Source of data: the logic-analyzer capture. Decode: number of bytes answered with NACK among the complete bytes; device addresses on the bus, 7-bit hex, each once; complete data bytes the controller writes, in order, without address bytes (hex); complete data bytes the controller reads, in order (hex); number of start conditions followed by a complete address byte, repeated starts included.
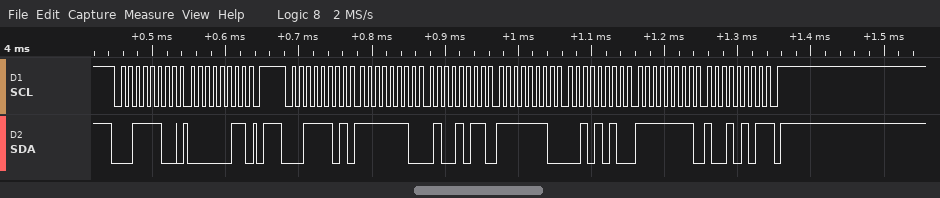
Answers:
1
0x1E
03
FE 4B FE 2A FF 95
2
